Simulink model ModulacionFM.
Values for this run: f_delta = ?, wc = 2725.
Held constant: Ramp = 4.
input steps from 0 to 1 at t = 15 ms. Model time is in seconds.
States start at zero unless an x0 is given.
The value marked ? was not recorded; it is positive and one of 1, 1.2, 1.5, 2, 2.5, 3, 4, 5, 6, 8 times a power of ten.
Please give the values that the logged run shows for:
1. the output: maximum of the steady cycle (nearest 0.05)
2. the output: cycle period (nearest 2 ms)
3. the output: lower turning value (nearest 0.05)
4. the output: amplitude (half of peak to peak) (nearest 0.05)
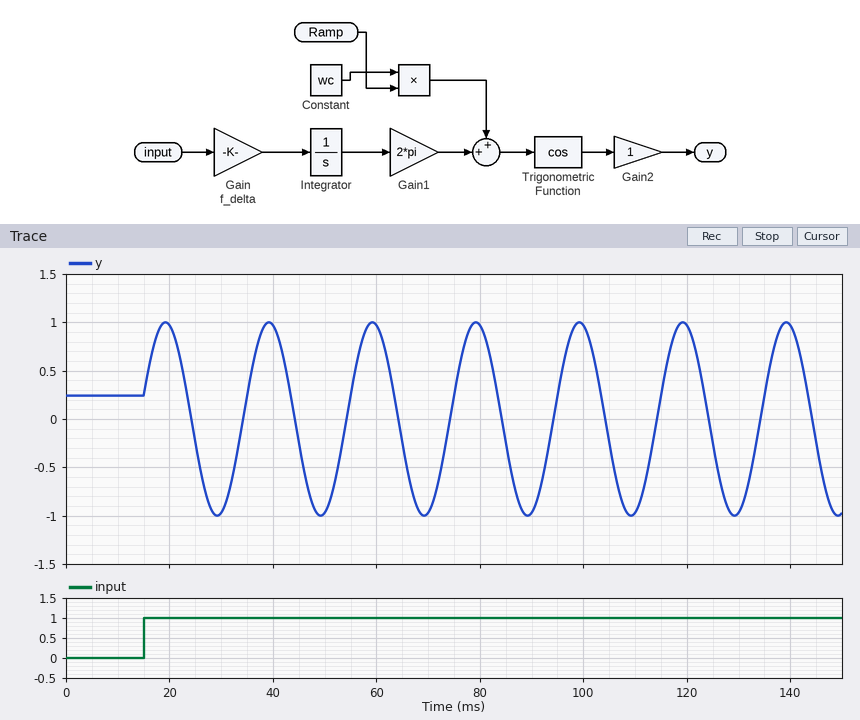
1.00
20 ms
-1.00
1.00
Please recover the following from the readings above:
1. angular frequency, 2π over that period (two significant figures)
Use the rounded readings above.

0.31 rad/ms
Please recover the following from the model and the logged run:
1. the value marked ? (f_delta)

50
